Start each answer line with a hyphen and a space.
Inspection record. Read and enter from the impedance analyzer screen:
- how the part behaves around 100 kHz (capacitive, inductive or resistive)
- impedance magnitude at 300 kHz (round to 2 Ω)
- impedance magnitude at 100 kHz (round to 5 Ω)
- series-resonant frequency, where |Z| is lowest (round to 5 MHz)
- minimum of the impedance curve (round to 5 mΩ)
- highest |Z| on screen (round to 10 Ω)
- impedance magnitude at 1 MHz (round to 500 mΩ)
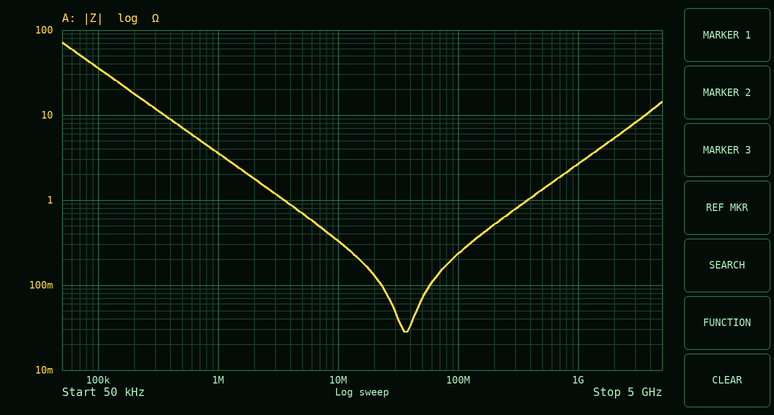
- capacitive
- 12 Ω
- 35 Ω
- 35 MHz
- 30 mΩ
- 70 Ω
- 3.5 Ω
